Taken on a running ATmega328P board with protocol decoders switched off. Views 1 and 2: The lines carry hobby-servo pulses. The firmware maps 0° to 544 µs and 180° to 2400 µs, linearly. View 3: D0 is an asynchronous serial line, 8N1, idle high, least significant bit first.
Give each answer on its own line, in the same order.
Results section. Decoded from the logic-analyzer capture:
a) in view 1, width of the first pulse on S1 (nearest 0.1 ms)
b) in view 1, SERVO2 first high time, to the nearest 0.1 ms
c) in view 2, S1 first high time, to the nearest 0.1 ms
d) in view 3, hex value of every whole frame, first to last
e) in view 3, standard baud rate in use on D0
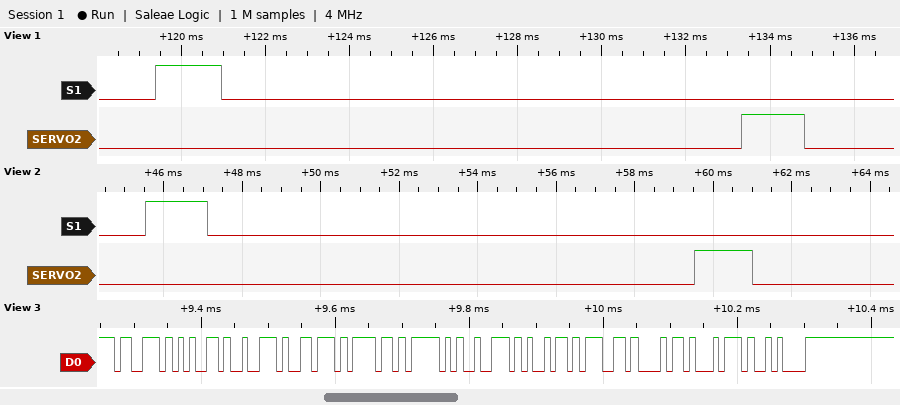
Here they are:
1.6 ms
1.5 ms
1.6 ms
73 65 72 76 6F 5F 72 69 67 68 74 0A
115200 baud
